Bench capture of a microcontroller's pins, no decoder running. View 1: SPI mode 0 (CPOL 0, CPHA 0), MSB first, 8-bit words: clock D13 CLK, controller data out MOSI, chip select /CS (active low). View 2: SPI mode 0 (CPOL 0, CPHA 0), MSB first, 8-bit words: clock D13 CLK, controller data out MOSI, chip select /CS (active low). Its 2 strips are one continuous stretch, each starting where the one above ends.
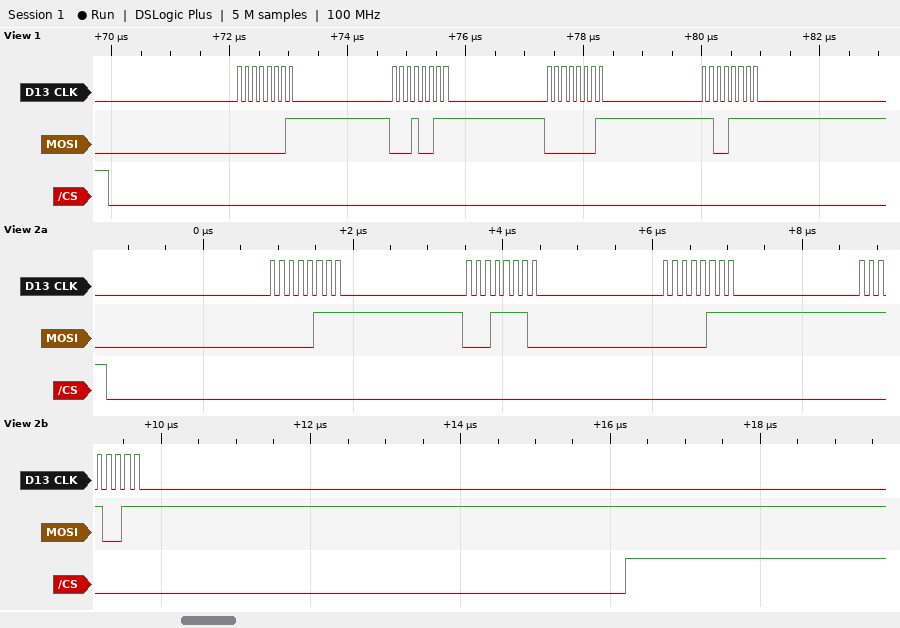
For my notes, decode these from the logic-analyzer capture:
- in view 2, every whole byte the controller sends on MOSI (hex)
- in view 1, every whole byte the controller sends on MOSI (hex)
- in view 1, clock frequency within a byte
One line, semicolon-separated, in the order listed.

07 1E 07 F3; 01 13 01 CF; 8 MHz
